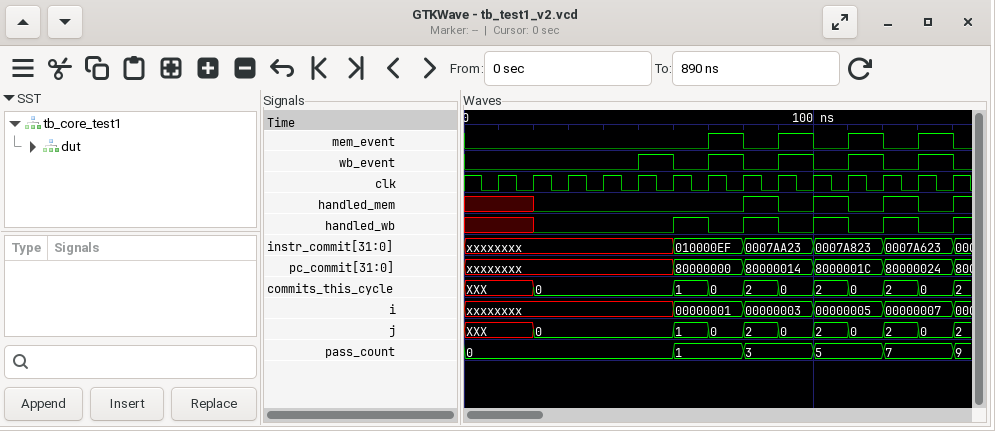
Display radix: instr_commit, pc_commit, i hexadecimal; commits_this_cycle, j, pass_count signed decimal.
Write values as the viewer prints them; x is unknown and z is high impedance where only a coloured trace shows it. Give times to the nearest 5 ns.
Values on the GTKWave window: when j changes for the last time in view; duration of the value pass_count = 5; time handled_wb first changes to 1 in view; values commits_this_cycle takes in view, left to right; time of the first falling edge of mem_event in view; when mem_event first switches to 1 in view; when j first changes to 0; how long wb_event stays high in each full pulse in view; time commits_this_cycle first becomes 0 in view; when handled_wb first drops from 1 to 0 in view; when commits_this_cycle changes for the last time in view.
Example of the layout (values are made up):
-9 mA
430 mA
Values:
140 ns
20 ns
60 ns
XXX, 0, 1, 0, 2, 0, 2, 0, 2, 0, 2
80 ns
70 ns
20 ns
10 ns, 10 ns, 10 ns, 10 ns, 10 ns
20 ns
70 ns
140 ns
